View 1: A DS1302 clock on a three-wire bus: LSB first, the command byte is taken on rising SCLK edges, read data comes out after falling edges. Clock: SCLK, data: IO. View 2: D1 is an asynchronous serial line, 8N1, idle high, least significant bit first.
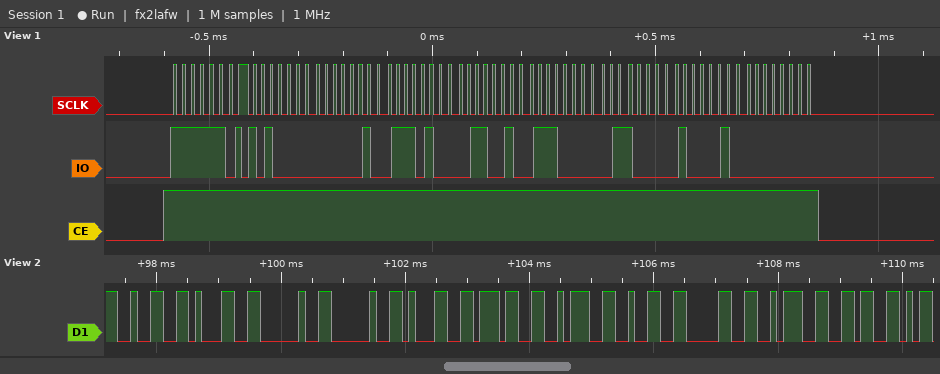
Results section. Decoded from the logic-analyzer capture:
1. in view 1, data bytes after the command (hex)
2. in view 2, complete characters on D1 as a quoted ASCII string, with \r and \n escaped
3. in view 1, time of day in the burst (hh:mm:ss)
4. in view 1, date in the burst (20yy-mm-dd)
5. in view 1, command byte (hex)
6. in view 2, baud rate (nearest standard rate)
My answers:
05 20 17 26 07 06 21 00
"21  17:20:6"
17:20:05
2021-07-26
0xBF
9600 baud
